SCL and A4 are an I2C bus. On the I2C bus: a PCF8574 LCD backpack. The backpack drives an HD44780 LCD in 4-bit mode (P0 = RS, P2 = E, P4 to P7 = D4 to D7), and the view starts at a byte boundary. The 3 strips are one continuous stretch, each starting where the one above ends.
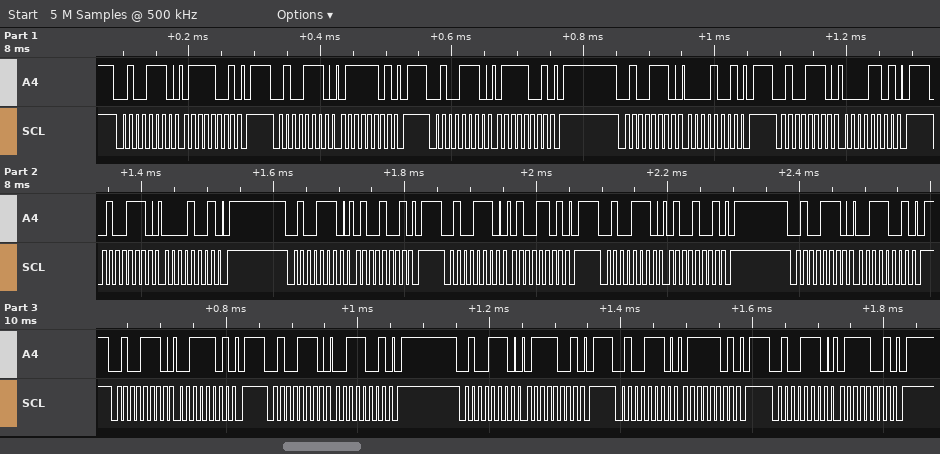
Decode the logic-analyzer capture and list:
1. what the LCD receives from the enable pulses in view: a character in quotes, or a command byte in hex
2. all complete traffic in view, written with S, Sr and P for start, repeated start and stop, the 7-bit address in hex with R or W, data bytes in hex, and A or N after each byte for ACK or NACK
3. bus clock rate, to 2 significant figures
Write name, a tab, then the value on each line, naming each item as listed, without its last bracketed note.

what the LCD receives from the enable pulses in view: a character in quotes, or a command byte in hex	'p' 'C'
all complete traffic in view, written with S, Sr and P for start, repeated start and stop, the 7-bit address in hex with R or W, data bytes in hex, and A or N after each byte for ACK or NACK	S 27W A 79 A P S 27W A 7D A P S 27W A 79 A P S 27W A 09 A P S 27W A 0D A P S 27W A 09 A P S 27W A 49 A P S 27W A 4D A P S 27W A 49 A P S 27W A 39 A P S 27W A 3D A P S 27W A 39 A P S 27W A 79 A P S 27W A 7D A P S 27W A 79 A P
bus clock rate, to 2 significant figures	100 kHz
